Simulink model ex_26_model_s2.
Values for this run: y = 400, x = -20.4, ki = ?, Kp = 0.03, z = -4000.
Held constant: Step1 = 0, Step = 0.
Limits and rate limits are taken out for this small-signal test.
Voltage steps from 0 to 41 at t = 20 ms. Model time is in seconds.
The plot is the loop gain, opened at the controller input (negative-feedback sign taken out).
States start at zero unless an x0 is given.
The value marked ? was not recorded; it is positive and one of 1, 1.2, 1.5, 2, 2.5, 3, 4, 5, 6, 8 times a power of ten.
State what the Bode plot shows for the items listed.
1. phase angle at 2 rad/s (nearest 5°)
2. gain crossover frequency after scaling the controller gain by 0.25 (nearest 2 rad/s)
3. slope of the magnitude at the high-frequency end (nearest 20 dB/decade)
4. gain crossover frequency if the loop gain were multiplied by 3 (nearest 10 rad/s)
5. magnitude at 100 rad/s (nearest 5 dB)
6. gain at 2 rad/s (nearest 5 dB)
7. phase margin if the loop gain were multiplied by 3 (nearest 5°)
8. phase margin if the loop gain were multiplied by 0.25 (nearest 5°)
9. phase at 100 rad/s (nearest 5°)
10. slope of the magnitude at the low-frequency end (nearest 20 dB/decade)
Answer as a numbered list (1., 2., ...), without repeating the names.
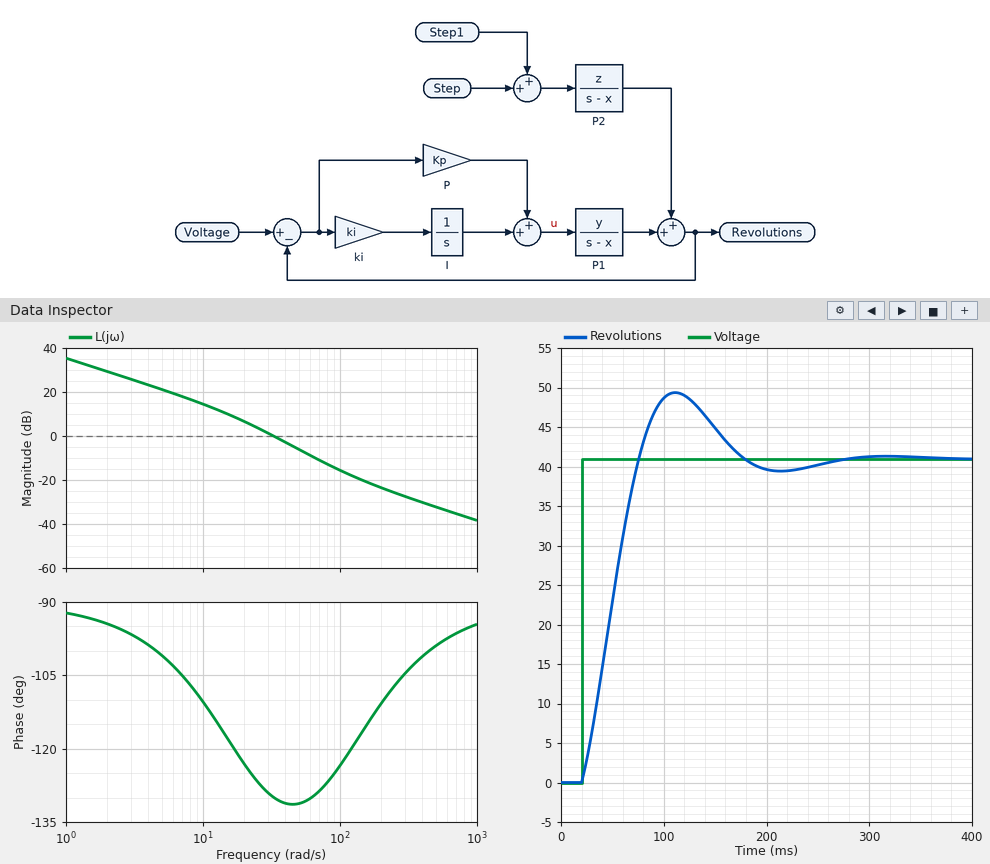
1. -95°
2. 12 rad/s
3. -20 dB/decade
4. 60 rad/s
5. -15 dB
6. 30 dB
7. 50°
8. 65°
9. -125°
10. -20 dB/decade
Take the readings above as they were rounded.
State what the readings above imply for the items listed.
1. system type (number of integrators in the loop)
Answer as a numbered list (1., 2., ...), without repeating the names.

1. 1
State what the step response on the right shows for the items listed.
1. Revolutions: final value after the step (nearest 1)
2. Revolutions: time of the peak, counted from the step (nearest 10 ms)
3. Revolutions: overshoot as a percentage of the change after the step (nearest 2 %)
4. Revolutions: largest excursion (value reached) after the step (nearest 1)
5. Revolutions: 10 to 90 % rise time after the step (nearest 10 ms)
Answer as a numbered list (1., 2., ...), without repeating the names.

1. 41
2. 90 ms
3. 20 %
4. 49
5. 40 ms
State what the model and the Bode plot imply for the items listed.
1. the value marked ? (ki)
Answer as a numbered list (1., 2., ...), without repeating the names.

1. 3
